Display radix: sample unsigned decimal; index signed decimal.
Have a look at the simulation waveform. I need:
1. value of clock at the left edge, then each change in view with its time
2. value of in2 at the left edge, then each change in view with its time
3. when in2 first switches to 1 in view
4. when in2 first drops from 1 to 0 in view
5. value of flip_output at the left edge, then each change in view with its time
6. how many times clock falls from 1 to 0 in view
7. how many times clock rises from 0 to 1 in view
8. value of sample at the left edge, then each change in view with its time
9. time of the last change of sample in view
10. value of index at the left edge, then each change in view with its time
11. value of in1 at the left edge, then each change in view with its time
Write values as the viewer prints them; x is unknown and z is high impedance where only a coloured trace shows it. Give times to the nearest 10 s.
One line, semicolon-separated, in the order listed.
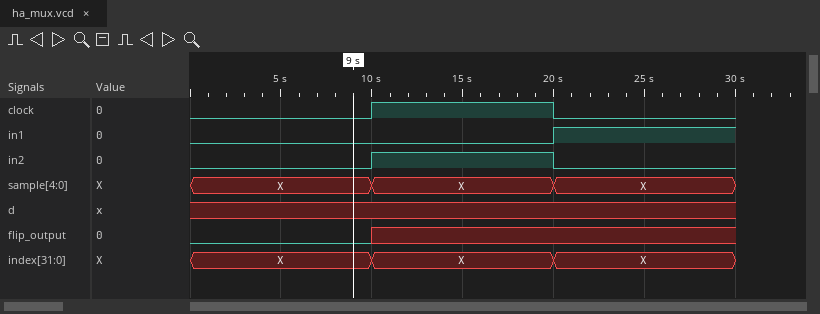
0, 1 at 10 s, 0 at 20 s; 0, 1 at 10 s, 0 at 20 s; 10 s; 20 s; 0, x at 10 s; 1; 1; X, X at 10 s, X at 20 s; 20 s; X, X at 10 s, X at 20 s; 0, 1 at 20 s
